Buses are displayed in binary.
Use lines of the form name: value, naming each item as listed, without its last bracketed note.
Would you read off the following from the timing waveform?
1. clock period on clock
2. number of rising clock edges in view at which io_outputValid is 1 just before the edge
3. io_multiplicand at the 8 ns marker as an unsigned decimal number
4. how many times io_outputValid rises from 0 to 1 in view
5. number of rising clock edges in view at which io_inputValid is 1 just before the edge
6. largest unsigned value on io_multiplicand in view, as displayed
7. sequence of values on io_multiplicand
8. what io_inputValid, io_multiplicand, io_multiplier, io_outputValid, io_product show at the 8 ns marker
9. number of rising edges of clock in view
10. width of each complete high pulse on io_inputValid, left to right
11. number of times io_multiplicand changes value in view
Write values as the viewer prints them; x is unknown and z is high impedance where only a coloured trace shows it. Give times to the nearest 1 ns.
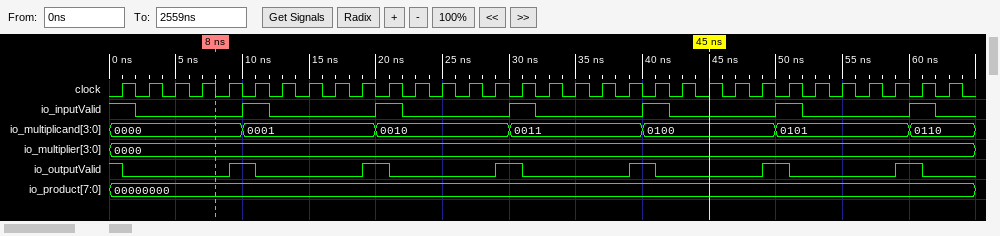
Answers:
clock period on clock: 2 ns
number of rising clock edges in view at which io_outputValid is 1 just before the edge: 7
io_multiplicand at the 8 ns marker as an unsigned decimal number: 0
how many times io_outputValid rises from 0 to 1 in view: 6
number of rising clock edges in view at which io_inputValid is 1 just before the edge: 7
largest unsigned value on io_multiplicand in view, as displayed: 0110
sequence of values on io_multiplicand: 0000, 0001, 0010, 0011, 0100, 0101, 0110
what io_inputValid, io_multiplicand, io_multiplier, io_outputValid, io_product show at the 8 ns marker: io_inputValid=0, io_multiplicand=0000, io_multiplier=0000, io_outputValid=0, io_product=00000000
number of rising edges of clock in view: 32
width of each complete high pulse on io_inputValid, left to right: 2 ns, 2 ns, 2 ns, 2 ns, 2 ns, 2 ns
number of times io_multiplicand changes value in view: 6
